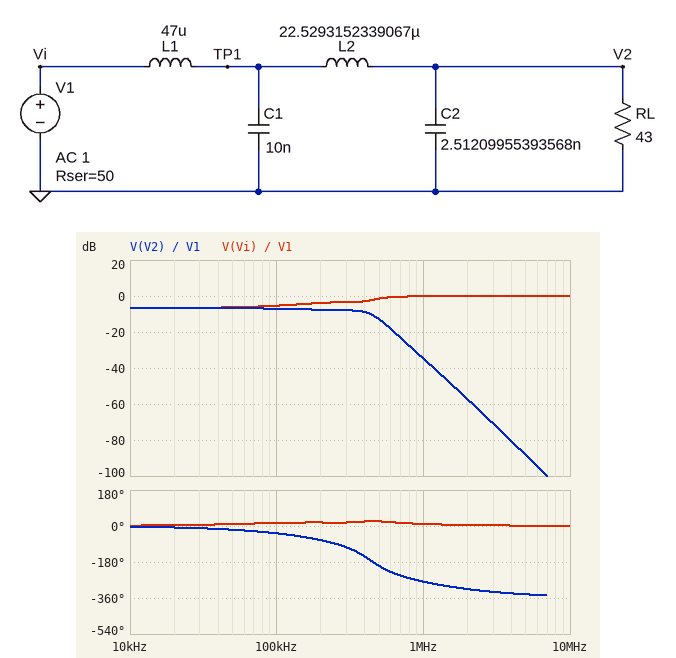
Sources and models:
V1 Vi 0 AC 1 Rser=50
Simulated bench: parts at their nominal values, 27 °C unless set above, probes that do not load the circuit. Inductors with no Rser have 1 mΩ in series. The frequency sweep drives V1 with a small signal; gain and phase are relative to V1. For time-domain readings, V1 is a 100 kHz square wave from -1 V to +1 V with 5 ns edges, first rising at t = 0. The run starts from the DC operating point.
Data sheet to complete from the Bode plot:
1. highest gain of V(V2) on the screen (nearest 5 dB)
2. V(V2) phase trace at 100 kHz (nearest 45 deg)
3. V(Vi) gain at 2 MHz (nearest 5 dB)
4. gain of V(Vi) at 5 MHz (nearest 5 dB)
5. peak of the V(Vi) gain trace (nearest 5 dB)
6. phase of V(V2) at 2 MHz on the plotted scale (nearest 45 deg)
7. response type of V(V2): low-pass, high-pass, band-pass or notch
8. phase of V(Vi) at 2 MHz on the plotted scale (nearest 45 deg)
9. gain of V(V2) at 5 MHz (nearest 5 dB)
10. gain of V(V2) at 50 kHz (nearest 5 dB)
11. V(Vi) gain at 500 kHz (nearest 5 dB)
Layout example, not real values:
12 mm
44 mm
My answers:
-5 dB
-45 deg
0 dB
0 dB
0 dB
-315 deg
low-pass
0 deg
-90 dB
-5 dB
0 dB
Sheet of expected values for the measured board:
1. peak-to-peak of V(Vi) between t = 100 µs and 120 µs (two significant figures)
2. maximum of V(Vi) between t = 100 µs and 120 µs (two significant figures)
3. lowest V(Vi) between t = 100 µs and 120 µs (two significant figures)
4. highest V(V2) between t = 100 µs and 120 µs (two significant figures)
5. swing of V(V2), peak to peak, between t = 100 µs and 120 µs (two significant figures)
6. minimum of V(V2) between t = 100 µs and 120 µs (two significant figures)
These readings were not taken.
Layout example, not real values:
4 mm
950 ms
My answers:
3.1 V
1.5 V
-1.5 V
500 mV
990 mV
-500 mV
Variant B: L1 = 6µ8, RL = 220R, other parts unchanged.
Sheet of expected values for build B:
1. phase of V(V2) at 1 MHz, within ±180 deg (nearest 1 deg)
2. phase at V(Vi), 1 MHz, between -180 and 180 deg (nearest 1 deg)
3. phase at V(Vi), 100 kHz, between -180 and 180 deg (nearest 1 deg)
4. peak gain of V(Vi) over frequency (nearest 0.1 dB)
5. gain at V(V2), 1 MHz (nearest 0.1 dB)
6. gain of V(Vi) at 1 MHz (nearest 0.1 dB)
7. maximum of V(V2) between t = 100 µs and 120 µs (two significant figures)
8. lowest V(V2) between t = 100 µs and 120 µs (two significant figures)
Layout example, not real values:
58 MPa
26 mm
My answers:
96 deg
63 deg
-17 deg
0 dB
-12.0 dB
-7.6 dB
970 mV
-970 mV
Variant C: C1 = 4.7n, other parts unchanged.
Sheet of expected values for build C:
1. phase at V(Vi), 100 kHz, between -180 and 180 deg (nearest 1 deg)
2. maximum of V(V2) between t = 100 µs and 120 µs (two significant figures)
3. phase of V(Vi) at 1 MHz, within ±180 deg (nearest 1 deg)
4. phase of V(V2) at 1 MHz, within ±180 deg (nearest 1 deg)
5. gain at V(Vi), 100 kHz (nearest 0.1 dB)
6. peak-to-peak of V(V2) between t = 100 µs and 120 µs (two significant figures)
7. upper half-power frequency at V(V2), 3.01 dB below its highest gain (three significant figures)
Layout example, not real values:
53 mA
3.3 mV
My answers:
18 deg
480 mV
11 deg
87 deg
-5.0 dB
950 mV
647 kHz
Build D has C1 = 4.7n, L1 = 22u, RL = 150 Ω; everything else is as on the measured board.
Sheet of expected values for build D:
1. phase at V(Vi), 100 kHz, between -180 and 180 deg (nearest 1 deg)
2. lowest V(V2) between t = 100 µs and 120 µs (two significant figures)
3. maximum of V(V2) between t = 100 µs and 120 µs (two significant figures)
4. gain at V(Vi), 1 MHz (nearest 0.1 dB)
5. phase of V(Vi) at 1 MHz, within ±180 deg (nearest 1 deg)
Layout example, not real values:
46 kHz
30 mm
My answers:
-7 deg
-1.1 V
1.1 V
-1.6 dB
29 deg
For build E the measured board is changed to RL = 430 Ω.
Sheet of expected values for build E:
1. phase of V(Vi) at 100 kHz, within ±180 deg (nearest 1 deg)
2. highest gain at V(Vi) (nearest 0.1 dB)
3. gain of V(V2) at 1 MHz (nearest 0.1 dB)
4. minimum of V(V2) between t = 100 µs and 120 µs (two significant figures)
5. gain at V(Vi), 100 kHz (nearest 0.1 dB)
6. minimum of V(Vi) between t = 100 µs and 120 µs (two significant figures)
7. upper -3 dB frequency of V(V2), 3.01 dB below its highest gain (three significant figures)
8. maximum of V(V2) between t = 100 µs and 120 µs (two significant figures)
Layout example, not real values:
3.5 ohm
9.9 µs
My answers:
-22 deg
0 dB
-25.1 dB
-1.3 V
-2.3 dB
-1.1 V
269 kHz
1.3 V
